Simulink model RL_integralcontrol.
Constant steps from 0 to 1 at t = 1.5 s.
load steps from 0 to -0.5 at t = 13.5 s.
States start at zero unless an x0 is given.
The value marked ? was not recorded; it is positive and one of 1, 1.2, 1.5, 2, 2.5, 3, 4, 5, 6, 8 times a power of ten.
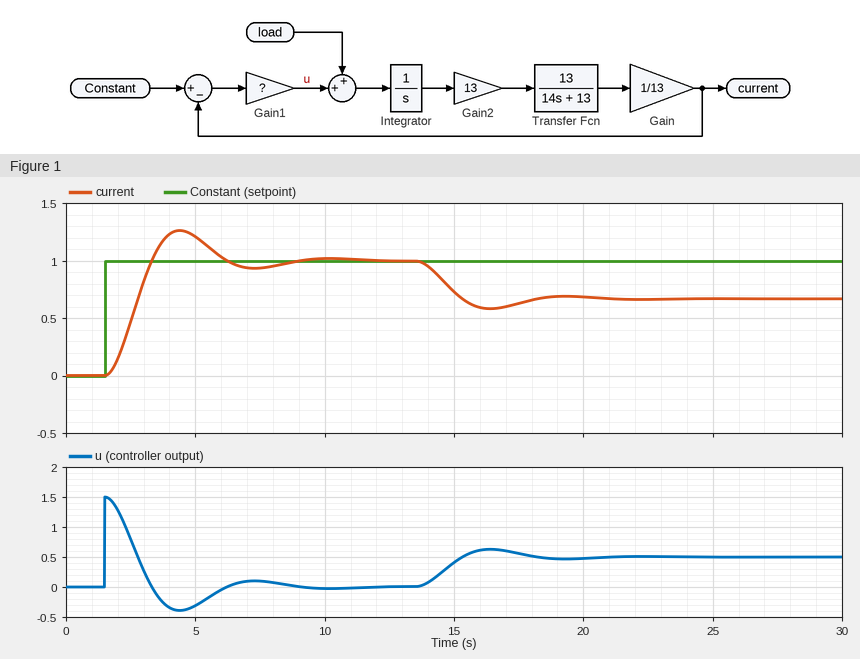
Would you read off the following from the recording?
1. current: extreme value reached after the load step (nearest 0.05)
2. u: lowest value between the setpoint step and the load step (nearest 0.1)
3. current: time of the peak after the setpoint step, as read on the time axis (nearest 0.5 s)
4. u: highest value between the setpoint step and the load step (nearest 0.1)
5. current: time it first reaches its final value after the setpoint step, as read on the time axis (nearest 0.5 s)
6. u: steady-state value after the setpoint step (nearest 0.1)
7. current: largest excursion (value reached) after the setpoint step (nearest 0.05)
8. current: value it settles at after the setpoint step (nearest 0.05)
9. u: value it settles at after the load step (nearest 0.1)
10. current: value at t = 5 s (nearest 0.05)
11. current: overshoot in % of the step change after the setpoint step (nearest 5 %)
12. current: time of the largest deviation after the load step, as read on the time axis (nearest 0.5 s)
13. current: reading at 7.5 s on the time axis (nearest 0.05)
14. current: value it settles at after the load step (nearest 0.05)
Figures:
0.60
-0.4
4.5 s
1.5
3.5 s
0.0
1.25
1.00
0.5
1.20
25 %
16.5 s
0.95
0.65
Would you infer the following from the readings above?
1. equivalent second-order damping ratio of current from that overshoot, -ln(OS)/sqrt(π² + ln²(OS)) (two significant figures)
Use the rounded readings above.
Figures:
0.40
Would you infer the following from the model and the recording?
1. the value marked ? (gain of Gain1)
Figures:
1.5
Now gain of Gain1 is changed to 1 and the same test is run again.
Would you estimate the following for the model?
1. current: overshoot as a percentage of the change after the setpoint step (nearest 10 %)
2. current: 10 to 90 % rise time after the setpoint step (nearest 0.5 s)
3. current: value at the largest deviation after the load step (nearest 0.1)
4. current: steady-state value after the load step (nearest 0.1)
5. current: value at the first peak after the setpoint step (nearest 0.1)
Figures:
20 %
1.5 s
0.4
0.5
1.2
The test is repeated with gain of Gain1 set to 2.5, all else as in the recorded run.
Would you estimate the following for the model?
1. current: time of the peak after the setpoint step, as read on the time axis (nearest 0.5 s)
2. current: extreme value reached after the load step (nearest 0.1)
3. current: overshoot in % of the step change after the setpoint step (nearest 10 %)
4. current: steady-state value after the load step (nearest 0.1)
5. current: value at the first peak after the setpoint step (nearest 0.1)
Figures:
3.5 s
0.7
40 %
0.8
1.4
